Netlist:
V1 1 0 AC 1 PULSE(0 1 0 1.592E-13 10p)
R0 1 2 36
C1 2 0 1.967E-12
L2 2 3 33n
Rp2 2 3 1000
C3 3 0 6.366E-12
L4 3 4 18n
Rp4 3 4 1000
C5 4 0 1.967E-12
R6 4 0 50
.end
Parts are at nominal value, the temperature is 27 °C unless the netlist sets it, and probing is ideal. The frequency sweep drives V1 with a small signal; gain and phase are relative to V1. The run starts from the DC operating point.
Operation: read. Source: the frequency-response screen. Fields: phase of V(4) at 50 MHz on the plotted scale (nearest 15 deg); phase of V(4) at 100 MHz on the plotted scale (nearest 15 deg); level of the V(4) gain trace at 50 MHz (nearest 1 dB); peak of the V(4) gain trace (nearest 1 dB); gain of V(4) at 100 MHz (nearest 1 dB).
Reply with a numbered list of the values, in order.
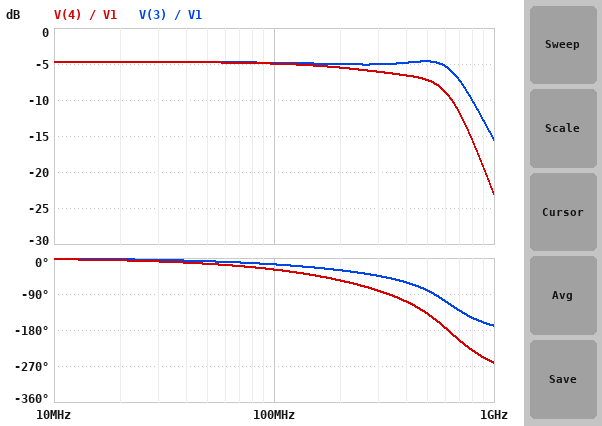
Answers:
1. -15 deg
2. -30 deg
3. -5 dB
4. -5 dB
5. -5 dB
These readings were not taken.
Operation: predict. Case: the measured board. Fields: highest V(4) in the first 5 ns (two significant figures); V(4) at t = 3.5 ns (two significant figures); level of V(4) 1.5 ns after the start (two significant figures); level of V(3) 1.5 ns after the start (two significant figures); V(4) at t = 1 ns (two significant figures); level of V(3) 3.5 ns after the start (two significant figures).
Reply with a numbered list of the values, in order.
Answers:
1. 590 mV
2. 580 mV
3. 590 mV
4. 570 mV
5. 440 mV
6. 580 mV
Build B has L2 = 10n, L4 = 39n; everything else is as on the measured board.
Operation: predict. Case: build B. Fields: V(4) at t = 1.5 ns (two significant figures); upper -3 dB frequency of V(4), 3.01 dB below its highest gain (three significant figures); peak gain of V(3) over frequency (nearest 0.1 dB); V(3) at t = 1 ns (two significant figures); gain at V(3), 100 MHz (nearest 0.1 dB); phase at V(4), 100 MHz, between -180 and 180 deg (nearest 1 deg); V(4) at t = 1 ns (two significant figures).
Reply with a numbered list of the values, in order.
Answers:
1. 550 mV
2. 421 MHz
3. 0.4 dB
4. 750 mV
5. -4.2 dB
6. -28 deg
7. 470 mV
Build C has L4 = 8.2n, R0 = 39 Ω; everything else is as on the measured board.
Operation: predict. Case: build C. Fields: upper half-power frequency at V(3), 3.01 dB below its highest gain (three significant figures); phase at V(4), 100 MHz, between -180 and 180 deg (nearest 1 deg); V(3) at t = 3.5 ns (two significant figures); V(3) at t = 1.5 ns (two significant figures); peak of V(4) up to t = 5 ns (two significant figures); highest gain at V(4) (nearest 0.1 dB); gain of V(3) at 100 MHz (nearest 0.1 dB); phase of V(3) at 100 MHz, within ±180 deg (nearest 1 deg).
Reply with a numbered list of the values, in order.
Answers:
1. 448 MHz
2. -25 deg
3. 560 mV
4. 570 mV
5. 570 mV
6. -5.0 dB
7. -5.1 dB
8. -19 deg
